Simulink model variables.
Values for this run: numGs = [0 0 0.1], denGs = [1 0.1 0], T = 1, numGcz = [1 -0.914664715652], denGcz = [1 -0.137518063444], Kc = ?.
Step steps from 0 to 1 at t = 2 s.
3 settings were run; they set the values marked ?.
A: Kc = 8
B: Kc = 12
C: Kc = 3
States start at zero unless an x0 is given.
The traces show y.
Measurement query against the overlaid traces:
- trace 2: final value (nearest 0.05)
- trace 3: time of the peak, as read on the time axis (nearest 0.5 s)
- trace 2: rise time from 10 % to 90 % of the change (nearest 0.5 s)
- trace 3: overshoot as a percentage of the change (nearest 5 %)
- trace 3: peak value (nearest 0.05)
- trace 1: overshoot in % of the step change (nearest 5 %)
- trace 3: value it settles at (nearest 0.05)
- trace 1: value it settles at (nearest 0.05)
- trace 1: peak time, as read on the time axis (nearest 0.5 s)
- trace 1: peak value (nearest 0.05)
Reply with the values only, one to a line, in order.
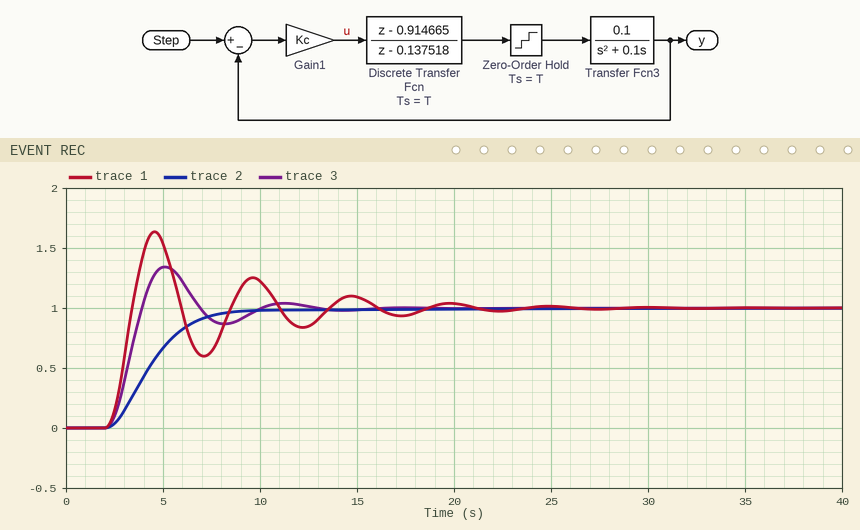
1.00
5.0 s
4.0 s
35 %
1.35
65 %
1.00
1.00
4.5 s
1.65
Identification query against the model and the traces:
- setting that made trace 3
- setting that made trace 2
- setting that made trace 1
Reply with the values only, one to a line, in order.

A
C
B
